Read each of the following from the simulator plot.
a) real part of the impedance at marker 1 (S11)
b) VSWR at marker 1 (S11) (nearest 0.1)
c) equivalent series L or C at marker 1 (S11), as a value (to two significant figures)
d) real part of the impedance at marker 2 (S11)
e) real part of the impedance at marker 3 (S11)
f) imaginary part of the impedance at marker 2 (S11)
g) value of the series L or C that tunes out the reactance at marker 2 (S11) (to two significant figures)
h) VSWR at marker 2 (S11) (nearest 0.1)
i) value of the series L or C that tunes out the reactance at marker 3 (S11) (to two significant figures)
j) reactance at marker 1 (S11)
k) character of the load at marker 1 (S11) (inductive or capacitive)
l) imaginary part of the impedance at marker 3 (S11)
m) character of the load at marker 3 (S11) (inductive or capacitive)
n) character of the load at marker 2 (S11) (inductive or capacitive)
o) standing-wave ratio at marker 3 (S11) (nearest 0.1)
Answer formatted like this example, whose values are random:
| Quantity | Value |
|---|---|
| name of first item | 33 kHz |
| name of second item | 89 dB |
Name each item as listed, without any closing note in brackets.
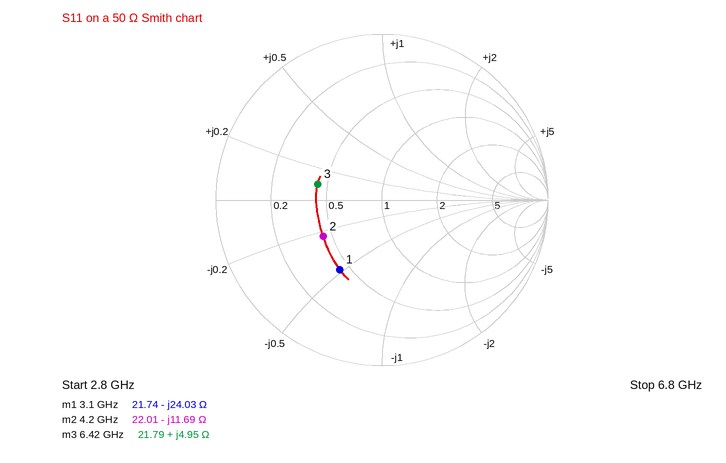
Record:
| Quantity | Value |
|---|---|
| real part of the impedance at marker 1 | 21.74 Ω |
| VSWR at marker 1 (S11) | 2.9 |
| equivalent series L or C at marker 1 (S11), as a value | 2.1 pF |
| real part of the impedance at marker 2 | 22.01 Ω |
| real part of the impedance at marker 3 | 21.79 Ω |
| imaginary part of the impedance at marker 2 | -11.69 Ω |
| value of the series L or C that tunes out the reactance at marker 2 (S11) | 440 pH |
| VSWR at marker 2 (S11) | 2.4 |
| value of the series L or C that tunes out the reactance at marker 3 (S11) | 5.0 pF |
| reactance at marker 1 | -24.03 Ω |
| character of the load at marker 1 (S11) | capacitive |
| imaginary part of the impedance at marker 3 | +4.95 Ω |
| character of the load at marker 3 (S11) | inductive |
| character of the load at marker 2 (S11) | capacitive |
| standing-wave ratio at marker 3 (S11) | 2.3 |
